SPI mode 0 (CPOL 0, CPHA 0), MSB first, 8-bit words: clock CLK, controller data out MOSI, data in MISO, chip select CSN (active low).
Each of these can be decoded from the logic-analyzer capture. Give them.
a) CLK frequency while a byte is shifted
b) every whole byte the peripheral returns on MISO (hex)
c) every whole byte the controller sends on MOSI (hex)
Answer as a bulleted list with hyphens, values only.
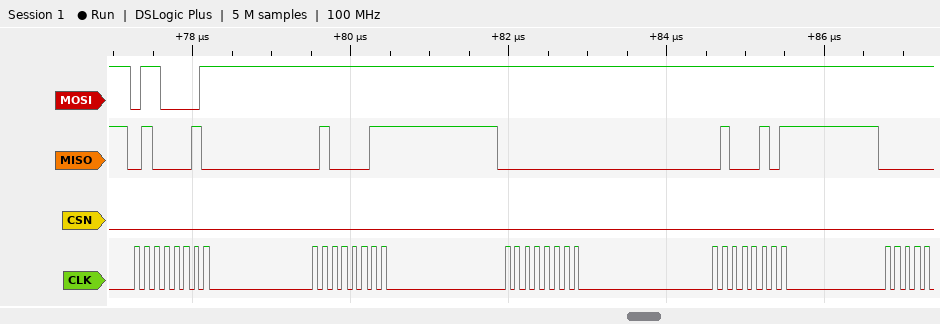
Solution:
- 8 MHz
- 42 43 00 45
- 61 FF FF FF
